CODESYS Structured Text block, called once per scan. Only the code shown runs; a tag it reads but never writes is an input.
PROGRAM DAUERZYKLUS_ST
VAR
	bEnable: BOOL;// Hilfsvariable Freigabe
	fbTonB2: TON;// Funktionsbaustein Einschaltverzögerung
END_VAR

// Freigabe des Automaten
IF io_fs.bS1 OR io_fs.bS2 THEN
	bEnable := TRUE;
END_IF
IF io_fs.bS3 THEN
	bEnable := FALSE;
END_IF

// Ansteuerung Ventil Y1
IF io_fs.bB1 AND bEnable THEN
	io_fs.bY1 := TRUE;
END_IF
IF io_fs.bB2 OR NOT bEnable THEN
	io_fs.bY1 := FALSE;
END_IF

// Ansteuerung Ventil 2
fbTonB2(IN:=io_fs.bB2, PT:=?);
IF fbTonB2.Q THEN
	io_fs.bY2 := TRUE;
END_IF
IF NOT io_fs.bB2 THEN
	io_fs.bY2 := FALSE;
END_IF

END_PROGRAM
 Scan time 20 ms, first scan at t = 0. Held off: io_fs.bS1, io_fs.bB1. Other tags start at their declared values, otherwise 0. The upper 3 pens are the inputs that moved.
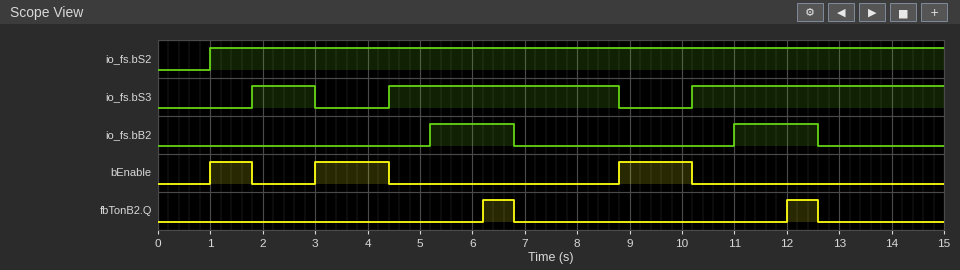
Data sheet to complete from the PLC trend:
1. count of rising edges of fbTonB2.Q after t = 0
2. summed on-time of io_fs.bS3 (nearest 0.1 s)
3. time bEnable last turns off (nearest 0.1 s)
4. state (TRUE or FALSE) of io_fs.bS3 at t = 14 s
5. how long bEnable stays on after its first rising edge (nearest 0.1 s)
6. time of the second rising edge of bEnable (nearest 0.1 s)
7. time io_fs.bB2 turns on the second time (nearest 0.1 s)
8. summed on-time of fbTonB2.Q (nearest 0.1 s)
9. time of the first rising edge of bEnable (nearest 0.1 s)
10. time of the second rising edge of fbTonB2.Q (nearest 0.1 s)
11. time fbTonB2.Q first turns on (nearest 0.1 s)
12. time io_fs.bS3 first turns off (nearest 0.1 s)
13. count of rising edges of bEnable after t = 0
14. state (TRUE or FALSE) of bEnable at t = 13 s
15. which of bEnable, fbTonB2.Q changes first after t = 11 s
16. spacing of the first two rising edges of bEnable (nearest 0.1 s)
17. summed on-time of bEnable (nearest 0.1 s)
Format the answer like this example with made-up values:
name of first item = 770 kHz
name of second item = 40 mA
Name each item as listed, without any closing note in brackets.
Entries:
count of rising edges of fbTonB2.Q after t = 0 = 2
summed on-time of io_fs.bS3 = 10.4 s
time bEnable last turns off = 10.2 s
state (TRUE or FALSE) of io_fs.bS3 at t = 14 s = TRUE
how long bEnable stays on after its first rising edge = 0.8 s
time of the second rising edge of bEnable = 3.0 s
time io_fs.bB2 turns on the second time = 11.0 s
summed on-time of fbTonB2.Q = 1.2 s
time of the first rising edge of bEnable = 1.0 s
time of the second rising edge of fbTonB2.Q = 12.0 s
time fbTonB2.Q first turns on = 6.2 s
time io_fs.bS3 first turns off = 3.0 s
count of rising edges of bEnable after t = 0 = 3
state (TRUE or FALSE) of bEnable at t = 13 s = FALSE
which of bEnable, fbTonB2.Q changes first after t = 11 s = fbTonB2.Q
spacing of the first two rising edges of bEnable = 2.0 s
summed on-time of bEnable = 3.6 s
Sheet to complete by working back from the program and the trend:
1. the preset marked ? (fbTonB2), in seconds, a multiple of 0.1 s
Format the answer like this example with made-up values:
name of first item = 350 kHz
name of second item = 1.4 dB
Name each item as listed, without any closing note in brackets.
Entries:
the preset marked ? (fbTonB2), in seconds, a multiple of 0.1 s = 1.0 s
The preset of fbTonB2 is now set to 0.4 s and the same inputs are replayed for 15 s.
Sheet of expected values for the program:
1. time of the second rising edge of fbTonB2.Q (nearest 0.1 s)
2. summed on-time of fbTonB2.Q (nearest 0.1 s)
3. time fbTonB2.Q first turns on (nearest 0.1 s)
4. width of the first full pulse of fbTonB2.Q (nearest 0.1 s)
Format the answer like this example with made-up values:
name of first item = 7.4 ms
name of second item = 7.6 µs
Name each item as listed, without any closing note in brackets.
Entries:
time of the second rising edge of fbTonB2.Q = 11.4 s
summed on-time of fbTonB2.Q = 2.4 s
time fbTonB2.Q first turns on = 5.6 s
width of the first full pulse of fbTonB2.Q = 1.2 s
